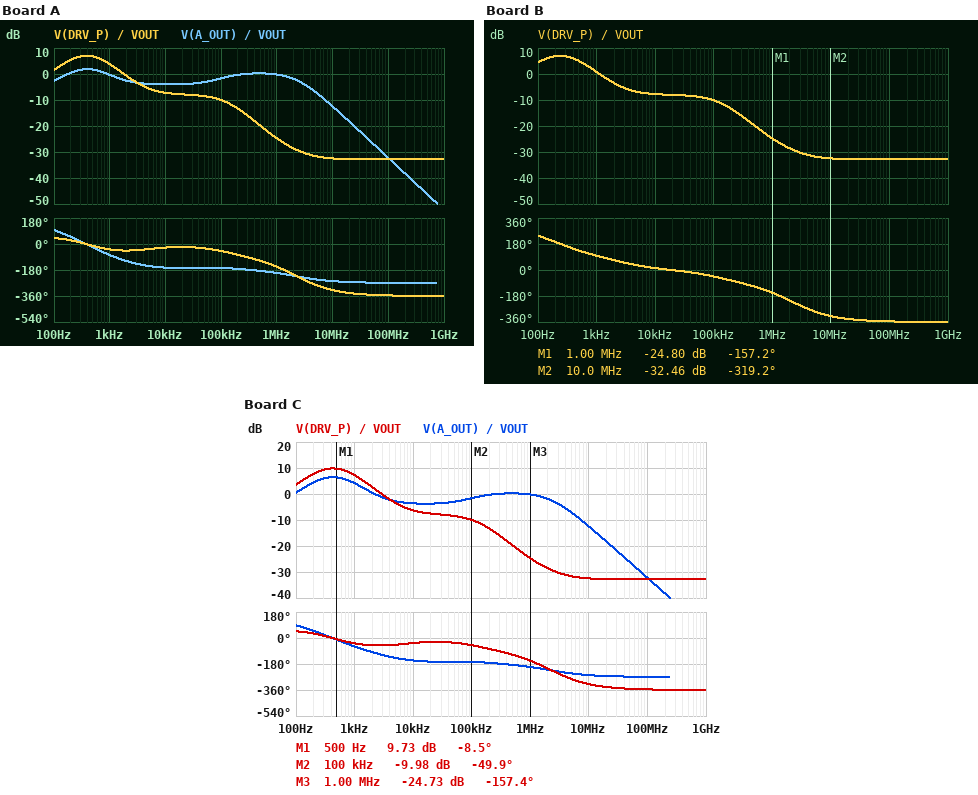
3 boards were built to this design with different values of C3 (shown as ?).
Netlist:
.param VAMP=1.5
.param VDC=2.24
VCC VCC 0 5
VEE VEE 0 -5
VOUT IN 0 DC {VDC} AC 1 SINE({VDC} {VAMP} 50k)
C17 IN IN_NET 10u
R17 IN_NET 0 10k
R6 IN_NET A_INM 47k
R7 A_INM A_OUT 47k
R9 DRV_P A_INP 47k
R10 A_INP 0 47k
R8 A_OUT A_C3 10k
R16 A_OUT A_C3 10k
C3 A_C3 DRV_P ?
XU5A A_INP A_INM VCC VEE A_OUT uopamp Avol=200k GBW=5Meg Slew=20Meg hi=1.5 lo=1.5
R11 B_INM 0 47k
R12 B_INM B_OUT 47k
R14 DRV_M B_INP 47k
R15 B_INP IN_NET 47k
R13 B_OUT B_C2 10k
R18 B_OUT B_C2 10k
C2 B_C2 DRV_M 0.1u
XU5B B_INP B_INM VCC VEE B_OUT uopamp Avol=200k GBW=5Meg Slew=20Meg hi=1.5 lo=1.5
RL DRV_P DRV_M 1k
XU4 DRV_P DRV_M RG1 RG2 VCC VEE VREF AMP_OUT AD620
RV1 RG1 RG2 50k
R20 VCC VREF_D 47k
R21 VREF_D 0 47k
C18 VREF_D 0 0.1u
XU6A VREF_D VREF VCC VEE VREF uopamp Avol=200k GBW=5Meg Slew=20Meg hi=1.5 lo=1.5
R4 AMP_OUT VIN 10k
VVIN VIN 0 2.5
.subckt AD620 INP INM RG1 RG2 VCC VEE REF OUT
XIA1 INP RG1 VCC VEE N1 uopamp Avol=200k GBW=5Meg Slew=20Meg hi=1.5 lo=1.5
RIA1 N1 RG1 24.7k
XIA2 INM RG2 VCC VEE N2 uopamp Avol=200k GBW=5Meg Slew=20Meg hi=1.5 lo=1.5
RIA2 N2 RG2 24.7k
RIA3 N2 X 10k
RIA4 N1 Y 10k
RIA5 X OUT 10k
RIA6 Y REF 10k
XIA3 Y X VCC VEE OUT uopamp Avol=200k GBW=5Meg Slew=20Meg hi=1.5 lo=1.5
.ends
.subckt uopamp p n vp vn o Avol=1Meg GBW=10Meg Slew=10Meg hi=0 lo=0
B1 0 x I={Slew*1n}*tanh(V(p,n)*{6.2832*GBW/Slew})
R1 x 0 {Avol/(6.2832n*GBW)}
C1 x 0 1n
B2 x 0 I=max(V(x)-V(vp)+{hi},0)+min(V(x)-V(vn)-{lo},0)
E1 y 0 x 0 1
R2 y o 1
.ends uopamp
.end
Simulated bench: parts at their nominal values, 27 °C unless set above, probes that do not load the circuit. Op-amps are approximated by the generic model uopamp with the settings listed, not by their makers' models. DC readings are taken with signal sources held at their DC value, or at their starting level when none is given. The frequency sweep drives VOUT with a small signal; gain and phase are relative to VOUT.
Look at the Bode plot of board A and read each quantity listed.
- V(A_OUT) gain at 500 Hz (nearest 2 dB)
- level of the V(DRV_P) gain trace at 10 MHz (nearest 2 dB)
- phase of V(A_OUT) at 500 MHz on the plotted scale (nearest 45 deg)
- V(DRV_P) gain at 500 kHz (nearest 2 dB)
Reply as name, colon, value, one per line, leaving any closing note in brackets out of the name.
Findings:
V(A_OUT) gain at 500 Hz: 2 dB
level of the V(DRV_P) gain trace at 10 MHz: -32 dB
phase of V(A_OUT) at 500 MHz on the plotted scale: -270 deg
V(DRV_P) gain at 500 kHz: -20 dB
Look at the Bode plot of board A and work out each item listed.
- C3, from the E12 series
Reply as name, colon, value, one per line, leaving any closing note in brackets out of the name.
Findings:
C3, from the E12 series: 68 nF
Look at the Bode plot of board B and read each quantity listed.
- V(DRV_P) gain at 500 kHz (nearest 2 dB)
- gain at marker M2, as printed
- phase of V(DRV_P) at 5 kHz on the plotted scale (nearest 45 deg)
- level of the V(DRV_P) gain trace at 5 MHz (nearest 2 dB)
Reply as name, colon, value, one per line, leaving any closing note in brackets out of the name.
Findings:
V(DRV_P) gain at 500 kHz: -20 dB
gain at marker M2, as printed: -32.46 dB
phase of V(DRV_P) at 5 kHz on the plotted scale: 45 deg
level of the V(DRV_P) gain trace at 5 MHz: -32 dB
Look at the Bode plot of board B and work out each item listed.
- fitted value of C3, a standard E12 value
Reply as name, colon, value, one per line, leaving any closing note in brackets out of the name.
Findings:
fitted value of C3, a standard E12 value: 180 nF
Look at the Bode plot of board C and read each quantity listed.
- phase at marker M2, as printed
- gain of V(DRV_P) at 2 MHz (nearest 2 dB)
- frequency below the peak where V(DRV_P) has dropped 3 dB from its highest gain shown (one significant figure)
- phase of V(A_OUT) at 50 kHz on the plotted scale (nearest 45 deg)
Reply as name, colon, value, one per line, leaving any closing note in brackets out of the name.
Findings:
phase at marker M2, as printed: -49.9 deg
gain of V(DRV_P) at 2 MHz: -28 dB
frequency below the peak where V(DRV_P) has dropped 3 dB from its highest gain shown: 200 Hz
phase of V(A_OUT) at 50 kHz on the plotted scale: -180 deg
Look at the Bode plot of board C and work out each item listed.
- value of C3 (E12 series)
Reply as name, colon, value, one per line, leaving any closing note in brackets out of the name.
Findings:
value of C3: 56 nF
